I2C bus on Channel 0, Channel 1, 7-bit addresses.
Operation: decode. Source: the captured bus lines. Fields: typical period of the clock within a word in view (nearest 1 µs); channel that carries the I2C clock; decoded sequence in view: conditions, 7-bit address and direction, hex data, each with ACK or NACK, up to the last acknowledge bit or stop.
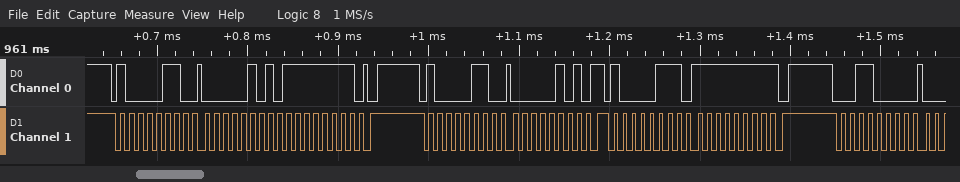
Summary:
10 µs
Channel 1
start, address 43 write ACK, 05 ACK, FF ACK, stop, start, address 43 write ACK, 05 ACK, repeated start, address 43 read ACK, FF NACK, stop, start, address 18 write ACK
